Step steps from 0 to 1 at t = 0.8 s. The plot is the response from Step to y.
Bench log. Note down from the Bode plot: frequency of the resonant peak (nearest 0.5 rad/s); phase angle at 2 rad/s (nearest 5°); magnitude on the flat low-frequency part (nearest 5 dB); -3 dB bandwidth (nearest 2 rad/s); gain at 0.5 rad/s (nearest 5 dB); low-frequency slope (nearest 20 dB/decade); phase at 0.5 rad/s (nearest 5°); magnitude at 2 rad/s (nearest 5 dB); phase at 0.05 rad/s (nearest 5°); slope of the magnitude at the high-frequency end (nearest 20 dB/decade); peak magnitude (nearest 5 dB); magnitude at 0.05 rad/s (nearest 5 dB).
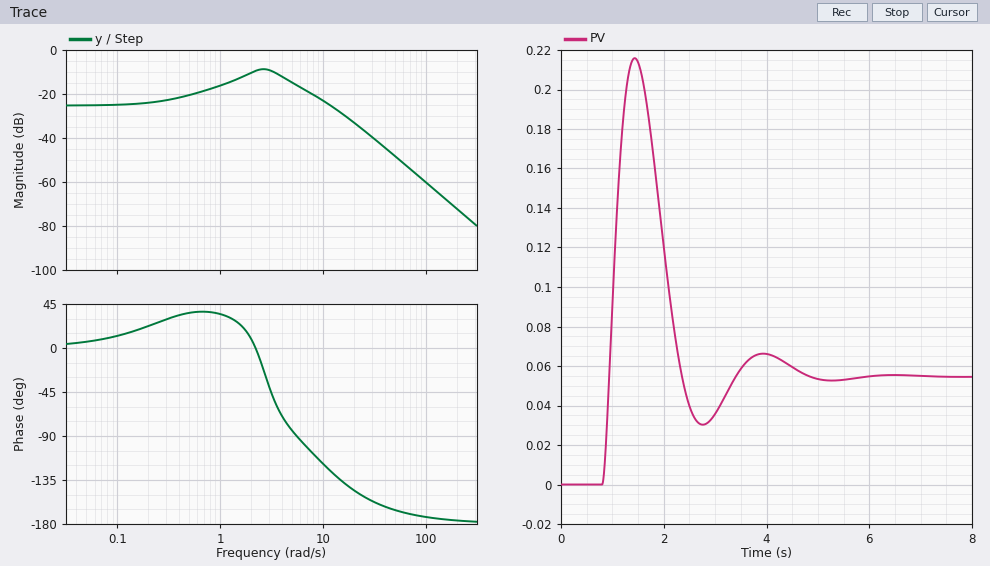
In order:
2.5 rad/s
10°
-25 dB
14 rad/s
-20 dB
0 dB/decade
35°
-10 dB
5°
-40 dB/decade
-10 dB
-25 dB
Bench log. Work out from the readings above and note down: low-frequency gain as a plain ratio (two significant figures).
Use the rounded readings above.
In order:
0.056
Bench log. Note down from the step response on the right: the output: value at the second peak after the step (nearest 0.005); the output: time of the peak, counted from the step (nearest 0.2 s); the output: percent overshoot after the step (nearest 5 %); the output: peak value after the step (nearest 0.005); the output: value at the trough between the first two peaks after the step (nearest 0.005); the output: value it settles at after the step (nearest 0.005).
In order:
0.065
0.6 s
295 %
0.215
0.030
0.055
